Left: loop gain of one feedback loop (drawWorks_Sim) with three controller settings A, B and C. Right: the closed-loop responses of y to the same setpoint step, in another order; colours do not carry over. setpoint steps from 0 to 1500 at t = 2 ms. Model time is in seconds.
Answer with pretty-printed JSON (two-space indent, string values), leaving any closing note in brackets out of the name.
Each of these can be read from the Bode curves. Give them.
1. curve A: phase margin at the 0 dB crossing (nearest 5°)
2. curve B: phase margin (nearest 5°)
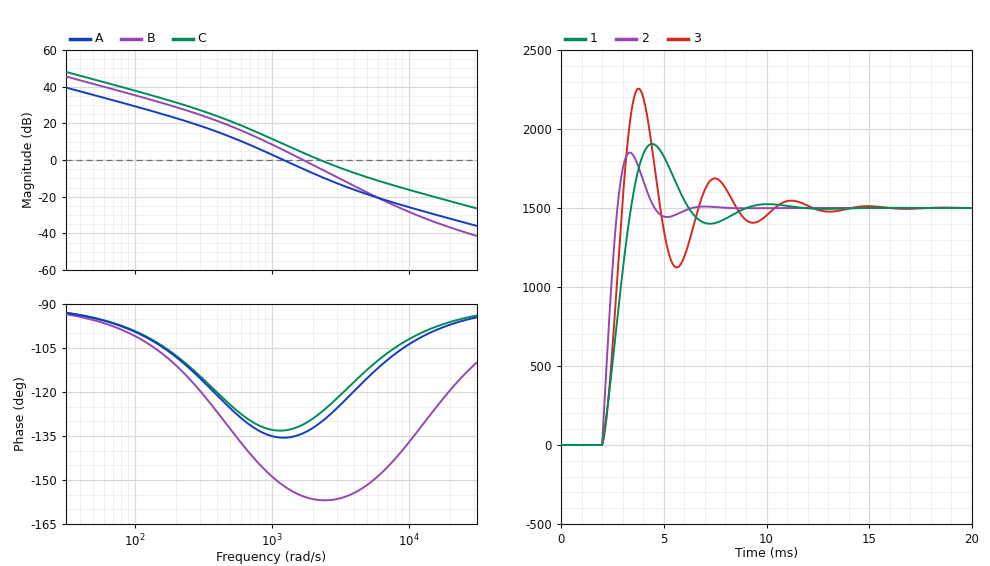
{
  "curve A: phase margin at the 0 dB crossing": "45°",
  "curve B: phase margin": "25°"
}
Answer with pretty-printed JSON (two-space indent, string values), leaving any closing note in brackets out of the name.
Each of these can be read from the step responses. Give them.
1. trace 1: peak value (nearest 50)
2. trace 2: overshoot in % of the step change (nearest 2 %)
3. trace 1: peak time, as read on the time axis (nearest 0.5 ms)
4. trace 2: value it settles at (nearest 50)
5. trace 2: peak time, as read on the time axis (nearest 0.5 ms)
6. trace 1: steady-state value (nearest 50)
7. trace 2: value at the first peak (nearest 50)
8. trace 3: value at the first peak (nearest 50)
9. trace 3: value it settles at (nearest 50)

{
  "trace 1: peak value": "1900",
  "trace 2: overshoot in % of the step change": "24 %",
  "trace 1: peak time, as read on the time axis": "4.5 ms",
  "trace 2: value it settles at": "1500",
  "trace 2: peak time, as read on the time axis": "3.5 ms",
  "trace 1: steady-state value": "1500",
  "trace 2: value at the first peak": "1850",
  "trace 3: value at the first peak": "2250",
  "trace 3: value it settles at": "1500"
}
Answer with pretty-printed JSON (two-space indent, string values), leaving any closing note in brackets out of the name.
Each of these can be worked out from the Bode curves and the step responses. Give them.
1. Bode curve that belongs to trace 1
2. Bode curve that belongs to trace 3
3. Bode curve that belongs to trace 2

{
  "Bode curve that belongs to trace 1": "A",
  "Bode curve that belongs to trace 3": "B",
  "Bode curve that belongs to trace 2": "C"
}
